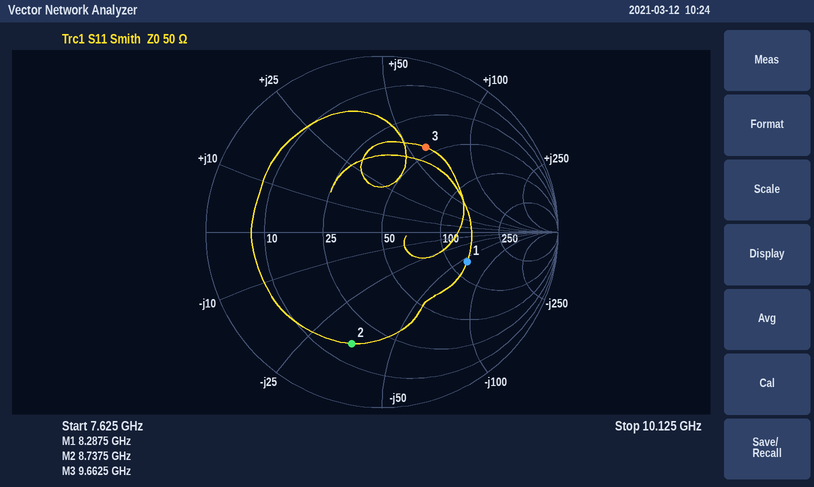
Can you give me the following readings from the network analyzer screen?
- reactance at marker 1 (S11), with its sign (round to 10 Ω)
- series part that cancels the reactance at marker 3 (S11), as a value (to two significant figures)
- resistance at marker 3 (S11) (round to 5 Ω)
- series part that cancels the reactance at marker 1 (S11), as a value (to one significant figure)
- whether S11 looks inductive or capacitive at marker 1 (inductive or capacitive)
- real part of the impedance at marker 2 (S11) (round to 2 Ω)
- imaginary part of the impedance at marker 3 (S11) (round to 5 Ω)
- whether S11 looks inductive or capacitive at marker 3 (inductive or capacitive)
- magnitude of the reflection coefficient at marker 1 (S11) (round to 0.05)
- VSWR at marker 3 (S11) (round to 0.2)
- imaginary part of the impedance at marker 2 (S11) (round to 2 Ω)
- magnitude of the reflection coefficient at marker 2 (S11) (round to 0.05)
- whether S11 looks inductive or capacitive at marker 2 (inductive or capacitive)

-60 Ω
270 fF
45 Ω
1 nH
capacitive
16 Ω
+60 Ω
inductive
0.50
3.4
-36 Ω
0.65
capacitive
